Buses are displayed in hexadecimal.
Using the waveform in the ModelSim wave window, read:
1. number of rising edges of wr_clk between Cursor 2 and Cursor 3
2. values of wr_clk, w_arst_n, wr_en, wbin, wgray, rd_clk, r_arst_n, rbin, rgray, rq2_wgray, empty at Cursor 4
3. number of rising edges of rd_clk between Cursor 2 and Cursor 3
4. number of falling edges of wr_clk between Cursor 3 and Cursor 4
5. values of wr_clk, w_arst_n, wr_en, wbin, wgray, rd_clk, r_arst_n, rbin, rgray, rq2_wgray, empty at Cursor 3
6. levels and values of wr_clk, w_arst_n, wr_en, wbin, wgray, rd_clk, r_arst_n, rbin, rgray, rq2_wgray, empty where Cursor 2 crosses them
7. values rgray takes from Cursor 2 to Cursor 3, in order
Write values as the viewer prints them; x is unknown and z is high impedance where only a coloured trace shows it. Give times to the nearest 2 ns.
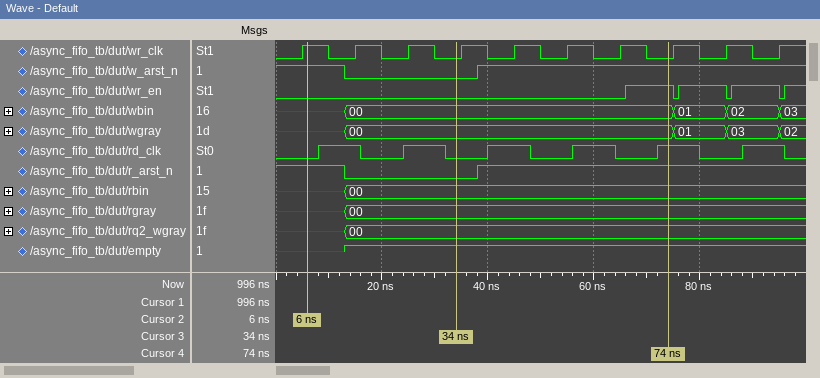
2
wr_clk=0, w_arst_n=1, wr_en=1, wbin=00, wgray=00, rd_clk=1, r_arst_n=1, rbin=00, rgray=00, rq2_wgray=00, empty=1
2
4
wr_clk=0, w_arst_n=0, wr_en=0, wbin=00, wgray=00, rd_clk=0, r_arst_n=0, rbin=00, rgray=00, rq2_wgray=00, empty=1
wr_clk=1, w_arst_n=1, wr_en=0, wbin=x, wgray=x, rd_clk=0, r_arst_n=1, rbin=x, rgray=x, rq2_wgray=x, empty=x
x, 00
